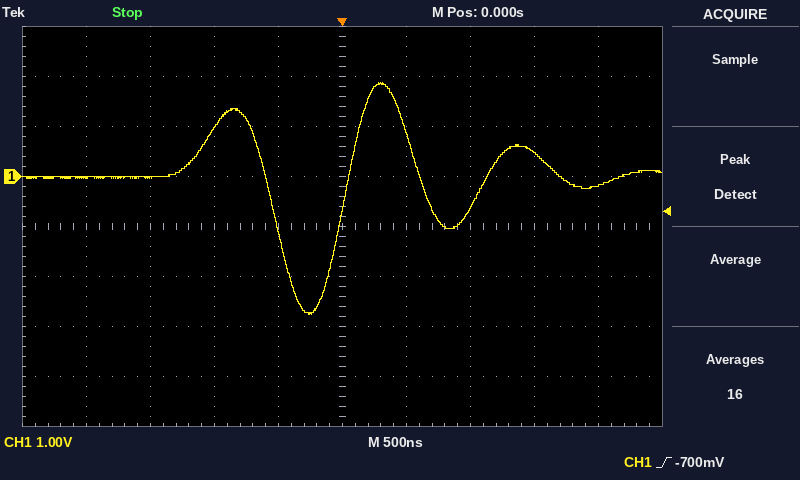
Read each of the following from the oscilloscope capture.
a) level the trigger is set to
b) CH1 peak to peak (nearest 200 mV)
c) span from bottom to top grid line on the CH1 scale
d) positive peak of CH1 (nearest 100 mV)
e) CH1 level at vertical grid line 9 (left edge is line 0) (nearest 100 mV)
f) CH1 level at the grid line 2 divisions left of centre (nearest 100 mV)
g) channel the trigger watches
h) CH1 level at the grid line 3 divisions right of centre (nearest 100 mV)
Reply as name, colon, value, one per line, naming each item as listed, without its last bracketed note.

level the trigger is set to: -700 mV
CH1 peak to peak: 4.6 V
span from bottom to top grid line on the CH1 scale: 8 V
positive peak of CH1: 1.9 V
CH1 level at vertical grid line 9 (left edge is line 0): -200 mV
CH1 level at the grid line 2 divisions left of centre: 1.0 V
channel the trigger watches: CH1
CH1 level at the grid line 3 divisions right of centre: 500 mV
